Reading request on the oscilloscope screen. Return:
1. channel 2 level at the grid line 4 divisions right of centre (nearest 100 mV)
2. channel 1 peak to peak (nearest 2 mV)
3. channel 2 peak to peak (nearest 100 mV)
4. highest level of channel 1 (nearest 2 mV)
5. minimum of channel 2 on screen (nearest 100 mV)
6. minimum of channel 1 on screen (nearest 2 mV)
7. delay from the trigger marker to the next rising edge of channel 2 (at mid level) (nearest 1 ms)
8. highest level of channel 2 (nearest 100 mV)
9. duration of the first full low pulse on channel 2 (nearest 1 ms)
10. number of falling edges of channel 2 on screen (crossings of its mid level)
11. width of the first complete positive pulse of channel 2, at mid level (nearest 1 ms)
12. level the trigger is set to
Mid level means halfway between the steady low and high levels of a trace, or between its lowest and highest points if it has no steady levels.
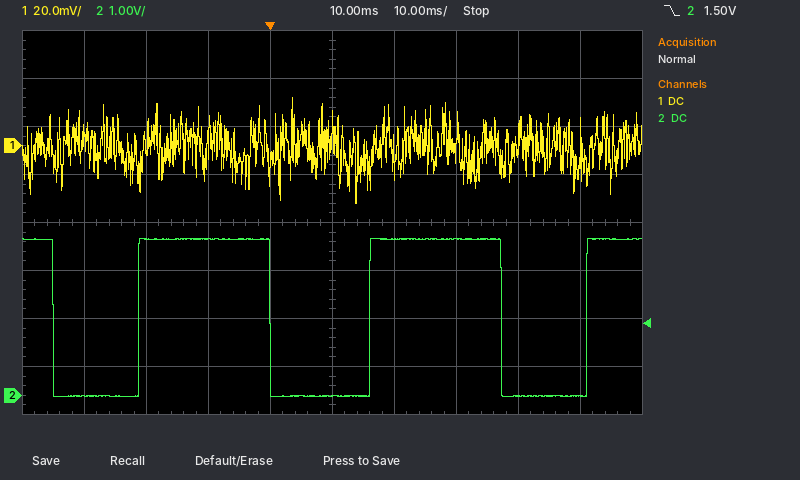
0.0 V
44 mV
3.3 V
20 mV
0.0 V
-24 mV
16 ms
3.3 V
14 ms
3
21 ms
1.50 V
